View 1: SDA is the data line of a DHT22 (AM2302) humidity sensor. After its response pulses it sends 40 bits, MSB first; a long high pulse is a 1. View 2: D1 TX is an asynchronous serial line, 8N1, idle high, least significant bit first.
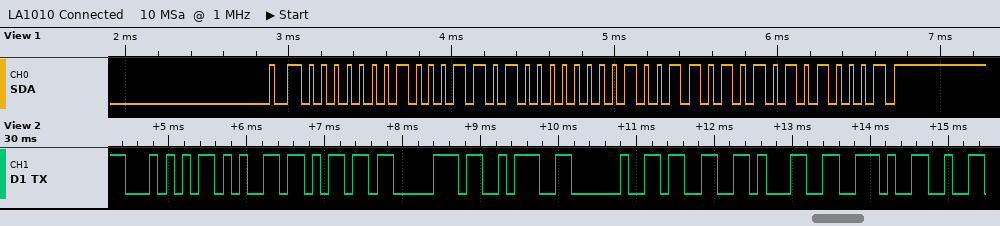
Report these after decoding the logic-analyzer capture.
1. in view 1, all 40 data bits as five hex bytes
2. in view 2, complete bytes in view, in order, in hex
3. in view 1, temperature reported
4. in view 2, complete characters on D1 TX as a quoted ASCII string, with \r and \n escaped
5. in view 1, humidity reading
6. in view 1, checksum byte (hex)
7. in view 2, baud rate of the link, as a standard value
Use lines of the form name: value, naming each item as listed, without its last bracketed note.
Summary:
in view 1, all 40 data bits as five hex bytes: 01 1A 01 35 51
in view 2, complete bytes in view, in order, in hex: 54 65 6D 70 3A 20 33 31 2E
in view 1, temperature reported: 30.9 °C
in view 2, complete characters on D1 TX as a quoted ASCII string, with \r and \n escaped: "Temp: 31."
in view 1, humidity reading: 28.2 %
in view 1, checksum byte: 0x51
in view 2, baud rate of the link, as a standard value: 9600 baud
